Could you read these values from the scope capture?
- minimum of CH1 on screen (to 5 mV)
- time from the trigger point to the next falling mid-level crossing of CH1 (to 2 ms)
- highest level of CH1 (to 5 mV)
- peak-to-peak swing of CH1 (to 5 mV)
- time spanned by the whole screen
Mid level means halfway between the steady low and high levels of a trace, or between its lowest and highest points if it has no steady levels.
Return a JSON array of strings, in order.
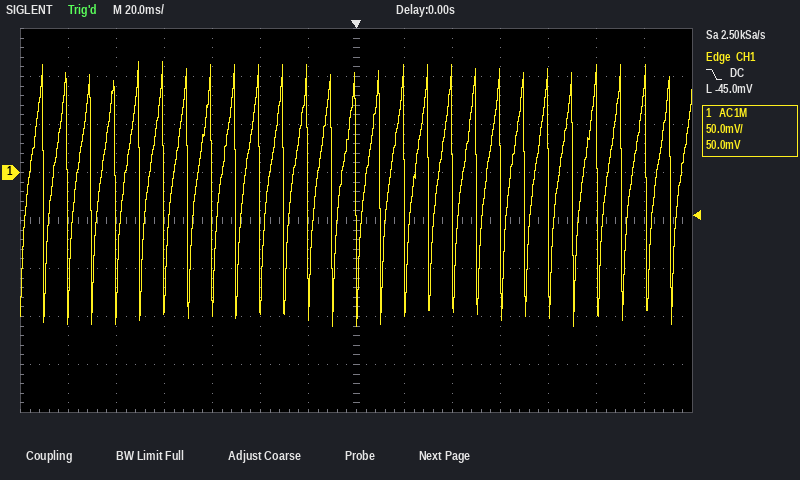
["-160 mV", "10 ms", "115 mV", "275 mV", "280 ms"]
